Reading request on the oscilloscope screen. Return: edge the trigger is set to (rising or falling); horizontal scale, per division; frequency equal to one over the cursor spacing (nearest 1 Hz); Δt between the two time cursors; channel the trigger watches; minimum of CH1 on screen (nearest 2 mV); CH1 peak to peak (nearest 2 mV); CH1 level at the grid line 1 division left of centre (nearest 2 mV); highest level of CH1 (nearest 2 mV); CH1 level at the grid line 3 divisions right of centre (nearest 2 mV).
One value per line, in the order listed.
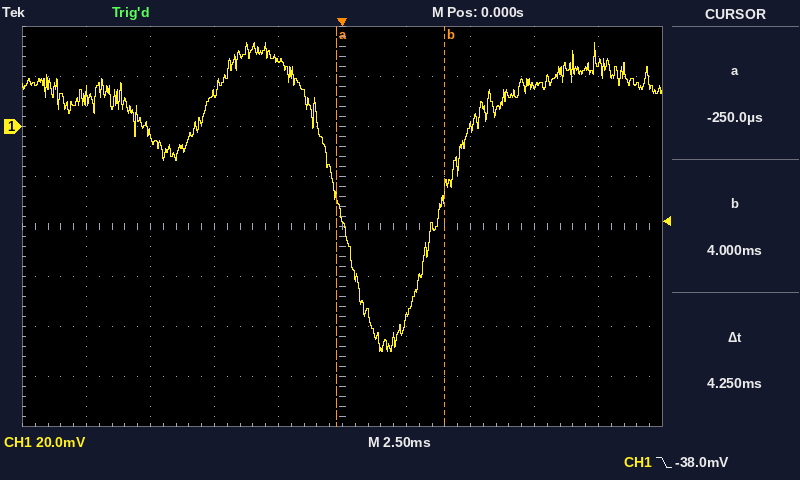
falling
2.5 ms
235 Hz
4.25 ms
CH1
-90 mV
124 mV
26 mV
34 mV
16 mV
